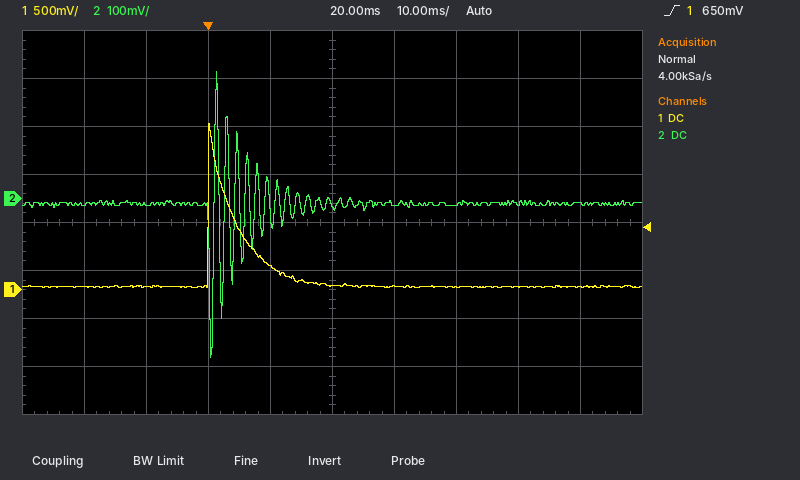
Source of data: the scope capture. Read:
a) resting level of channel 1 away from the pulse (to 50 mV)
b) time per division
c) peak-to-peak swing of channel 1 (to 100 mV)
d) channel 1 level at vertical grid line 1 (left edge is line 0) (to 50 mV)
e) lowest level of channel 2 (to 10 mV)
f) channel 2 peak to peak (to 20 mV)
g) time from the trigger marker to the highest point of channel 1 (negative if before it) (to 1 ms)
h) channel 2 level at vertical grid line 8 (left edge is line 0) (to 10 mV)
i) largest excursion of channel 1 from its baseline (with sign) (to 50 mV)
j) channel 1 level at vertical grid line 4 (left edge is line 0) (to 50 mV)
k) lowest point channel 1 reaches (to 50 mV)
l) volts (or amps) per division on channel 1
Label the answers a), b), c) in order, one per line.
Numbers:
a) 50 mV
b) 10 ms
c) 1.70 V
d) 50 mV
e) -330 mV
f) 600 mV
g) 0 ms
h) -10 mV
i) +1.70 V
j) 250 mV
k) 0 mV
l) 500 mV
